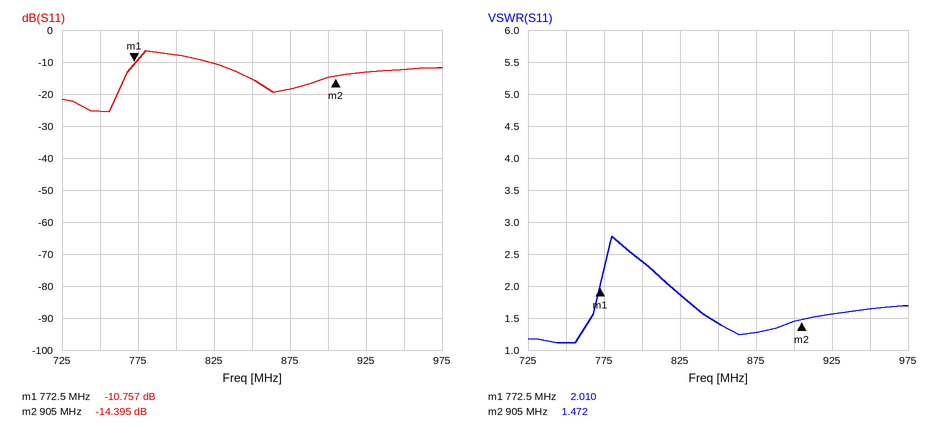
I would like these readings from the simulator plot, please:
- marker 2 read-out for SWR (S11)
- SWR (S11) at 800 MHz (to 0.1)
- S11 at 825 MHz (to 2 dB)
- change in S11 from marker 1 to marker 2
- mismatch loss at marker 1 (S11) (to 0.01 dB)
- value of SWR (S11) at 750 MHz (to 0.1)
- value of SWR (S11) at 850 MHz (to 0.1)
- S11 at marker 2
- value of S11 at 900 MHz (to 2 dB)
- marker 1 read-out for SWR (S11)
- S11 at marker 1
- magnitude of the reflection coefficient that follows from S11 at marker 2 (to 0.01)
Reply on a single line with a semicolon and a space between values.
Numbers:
1.472; 2.4; -10 dB; -3.638 dB; 0.38 dB; 1.1; 1.4; -14.395 dB; -14 dB; 2.010; -10.757 dB; 0.19
